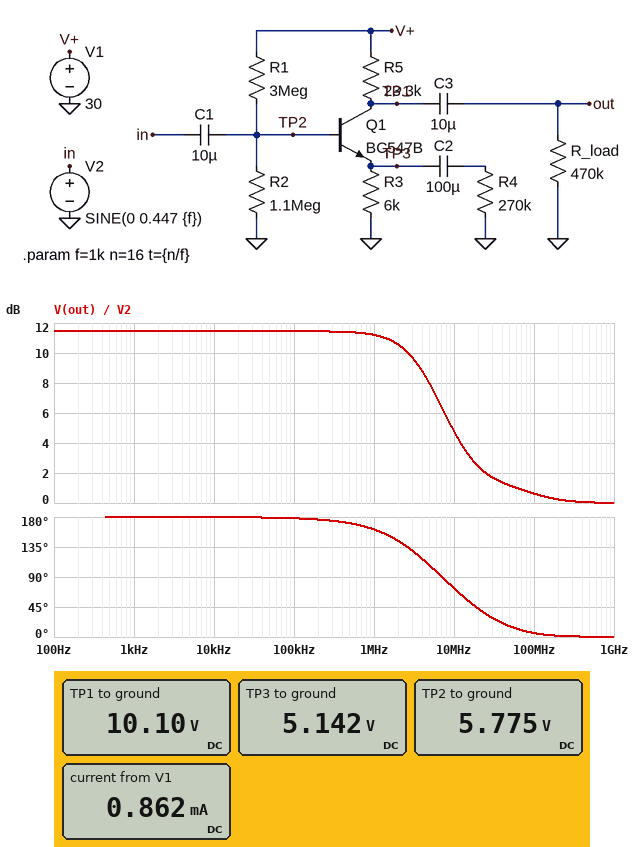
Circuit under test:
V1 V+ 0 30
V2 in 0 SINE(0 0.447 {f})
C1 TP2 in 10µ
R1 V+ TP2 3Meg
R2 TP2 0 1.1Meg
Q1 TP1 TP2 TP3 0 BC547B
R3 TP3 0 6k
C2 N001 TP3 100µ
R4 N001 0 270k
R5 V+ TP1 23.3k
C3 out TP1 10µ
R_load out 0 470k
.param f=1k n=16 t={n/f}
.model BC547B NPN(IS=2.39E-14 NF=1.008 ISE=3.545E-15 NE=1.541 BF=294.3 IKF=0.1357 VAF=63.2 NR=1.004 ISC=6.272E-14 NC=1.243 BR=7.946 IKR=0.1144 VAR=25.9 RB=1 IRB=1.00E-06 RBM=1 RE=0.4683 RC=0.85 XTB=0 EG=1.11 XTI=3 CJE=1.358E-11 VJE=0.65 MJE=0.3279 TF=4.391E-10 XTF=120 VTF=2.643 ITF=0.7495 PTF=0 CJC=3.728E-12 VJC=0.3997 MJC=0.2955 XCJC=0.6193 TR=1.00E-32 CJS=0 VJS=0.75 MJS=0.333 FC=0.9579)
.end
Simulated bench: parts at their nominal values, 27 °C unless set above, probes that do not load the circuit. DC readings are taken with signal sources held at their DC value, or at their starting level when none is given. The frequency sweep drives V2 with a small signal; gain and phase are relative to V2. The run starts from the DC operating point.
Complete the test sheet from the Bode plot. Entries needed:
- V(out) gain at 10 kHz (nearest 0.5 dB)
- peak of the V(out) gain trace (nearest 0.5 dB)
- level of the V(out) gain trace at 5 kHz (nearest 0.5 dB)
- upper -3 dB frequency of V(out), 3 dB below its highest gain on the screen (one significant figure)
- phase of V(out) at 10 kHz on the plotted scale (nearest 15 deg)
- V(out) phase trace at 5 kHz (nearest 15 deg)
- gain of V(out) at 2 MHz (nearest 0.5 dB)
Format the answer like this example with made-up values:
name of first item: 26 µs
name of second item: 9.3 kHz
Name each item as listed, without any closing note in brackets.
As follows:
V(out) gain at 10 kHz: 11.5 dB
peak of the V(out) gain trace: 11.5 dB
level of the V(out) gain trace at 5 kHz: 11.5 dB
upper -3 dB frequency of V(out), 3 dB below its highest gain on the screen: 4 MHz
phase of V(out) at 10 kHz on the plotted scale: 180 deg
V(out) phase trace at 5 kHz: 180 deg
gain of V(out) at 2 MHz: 10.5 dB
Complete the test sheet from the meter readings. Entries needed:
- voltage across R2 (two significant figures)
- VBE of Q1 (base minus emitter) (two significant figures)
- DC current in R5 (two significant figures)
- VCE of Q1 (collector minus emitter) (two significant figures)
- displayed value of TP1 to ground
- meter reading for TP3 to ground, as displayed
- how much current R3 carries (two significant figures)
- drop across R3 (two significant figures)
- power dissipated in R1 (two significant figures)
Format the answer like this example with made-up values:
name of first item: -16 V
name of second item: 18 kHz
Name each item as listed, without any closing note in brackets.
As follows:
voltage across R2: 5.8 V
VBE of Q1 (base minus emitter): 630 mV
DC current in R5: 850 µA
VCE of Q1 (collector minus emitter): 5.0 V
displayed value of TP1 to ground: 10.10 V
meter reading for TP3 to ground, as displayed: 5.142 V
how much current R3 carries: 860 µA
drop across R3: 5.1 V
power dissipated in R1: 200 µW
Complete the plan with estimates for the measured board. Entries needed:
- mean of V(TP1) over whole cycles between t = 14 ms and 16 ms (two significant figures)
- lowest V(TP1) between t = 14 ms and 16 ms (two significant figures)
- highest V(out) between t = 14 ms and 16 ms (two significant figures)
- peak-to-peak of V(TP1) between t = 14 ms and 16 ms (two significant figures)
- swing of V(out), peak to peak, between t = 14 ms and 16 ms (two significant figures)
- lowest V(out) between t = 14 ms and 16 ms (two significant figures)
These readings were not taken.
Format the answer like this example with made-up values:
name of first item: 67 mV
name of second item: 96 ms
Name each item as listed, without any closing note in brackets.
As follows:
mean of V(TP1) over whole cycles between t = 14 ms and 16 ms: 10 V
lowest V(TP1) between t = 14 ms and 16 ms: 8.4 V
highest V(out) between t = 14 ms and 16 ms: 1.7 V
peak-to-peak of V(TP1) between t = 14 ms and 16 ms: 3.3 V
swing of V(out), peak to peak, between t = 14 ms and 16 ms: 3.3 V
lowest V(out) between t = 14 ms and 16 ms: -1.7 V
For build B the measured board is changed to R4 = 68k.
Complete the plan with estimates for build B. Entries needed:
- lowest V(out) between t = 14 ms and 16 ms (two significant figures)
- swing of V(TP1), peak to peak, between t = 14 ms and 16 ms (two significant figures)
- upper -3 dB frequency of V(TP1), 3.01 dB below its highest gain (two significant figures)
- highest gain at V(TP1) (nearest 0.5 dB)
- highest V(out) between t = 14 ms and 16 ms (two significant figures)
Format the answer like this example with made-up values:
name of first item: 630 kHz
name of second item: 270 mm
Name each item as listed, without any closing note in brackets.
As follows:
lowest V(out) between t = 14 ms and 16 ms: -1.8 V
swing of V(TP1), peak to peak, between t = 14 ms and 16 ms: 3.6 V
upper -3 dB frequency of V(TP1), 3.01 dB below its highest gain: 4.3 MHz
highest gain at V(TP1): 12.0 dB
highest V(out) between t = 14 ms and 16 ms: 1.8 V
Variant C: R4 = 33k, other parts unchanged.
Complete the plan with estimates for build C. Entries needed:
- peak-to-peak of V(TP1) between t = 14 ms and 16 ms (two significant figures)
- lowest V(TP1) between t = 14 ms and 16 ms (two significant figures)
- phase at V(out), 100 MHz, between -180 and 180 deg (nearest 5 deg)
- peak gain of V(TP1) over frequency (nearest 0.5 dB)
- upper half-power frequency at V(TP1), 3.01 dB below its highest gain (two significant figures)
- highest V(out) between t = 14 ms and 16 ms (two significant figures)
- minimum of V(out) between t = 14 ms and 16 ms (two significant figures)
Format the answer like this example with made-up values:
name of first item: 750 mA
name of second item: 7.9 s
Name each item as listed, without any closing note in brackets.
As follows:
peak-to-peak of V(TP1) between t = 14 ms and 16 ms: 3.9 V
lowest V(TP1) between t = 14 ms and 16 ms: 8.2 V
phase at V(out), 100 MHz, between -180 and 180 deg: 5 deg
peak gain of V(TP1) over frequency: 12.5 dB
upper half-power frequency at V(TP1), 3.01 dB below its highest gain: 4.3 MHz
highest V(out) between t = 14 ms and 16 ms: 1.9 V
minimum of V(out) between t = 14 ms and 16 ms: -1.9 V
